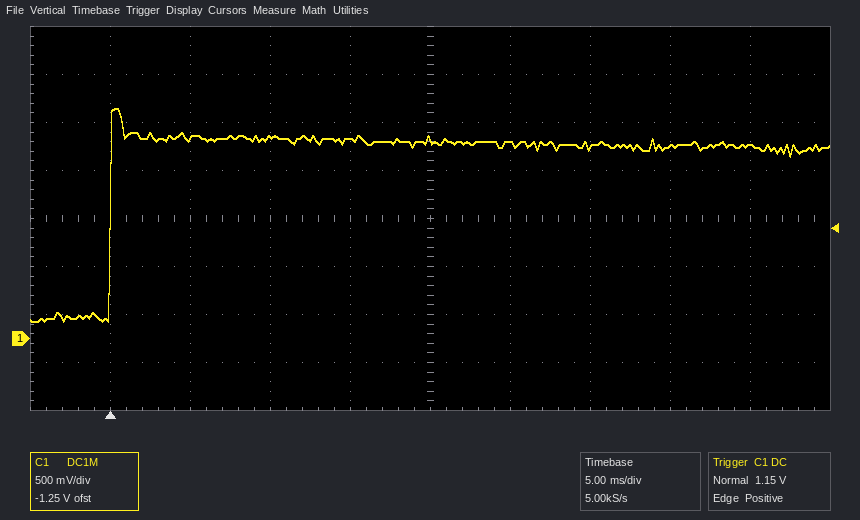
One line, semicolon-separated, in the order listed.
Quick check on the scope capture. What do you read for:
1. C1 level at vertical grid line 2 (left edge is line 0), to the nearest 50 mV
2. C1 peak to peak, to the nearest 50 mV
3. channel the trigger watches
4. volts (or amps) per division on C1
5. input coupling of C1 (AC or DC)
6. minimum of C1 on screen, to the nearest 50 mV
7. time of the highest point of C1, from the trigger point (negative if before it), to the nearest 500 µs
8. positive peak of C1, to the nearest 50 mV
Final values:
2.10 V; 2.20 V; C1; 500 mV; DC; 200 mV; +500 µs; 2.40 V
